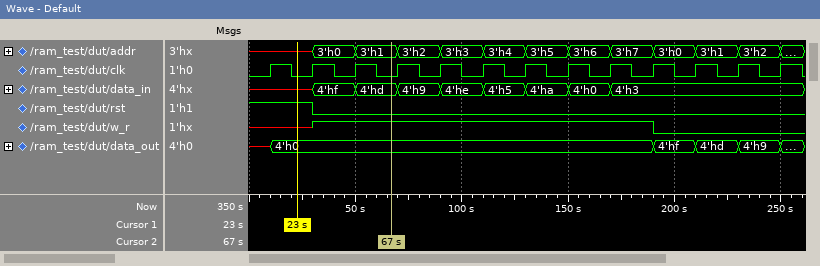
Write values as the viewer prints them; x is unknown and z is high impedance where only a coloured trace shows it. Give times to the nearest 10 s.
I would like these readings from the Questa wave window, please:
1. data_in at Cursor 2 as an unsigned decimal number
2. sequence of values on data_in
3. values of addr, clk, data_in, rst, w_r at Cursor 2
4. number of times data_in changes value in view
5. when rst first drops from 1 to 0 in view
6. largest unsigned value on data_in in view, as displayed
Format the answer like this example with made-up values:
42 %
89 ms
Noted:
13
x, 4'hf, 4'hd, 4'h9, 4'he, 4'h5, 4'ha, 4'h0, 4'h3
addr=3'h1, clk=0, data_in=4'hd, rst=0, w_r=1
8
30 s
4'hf
